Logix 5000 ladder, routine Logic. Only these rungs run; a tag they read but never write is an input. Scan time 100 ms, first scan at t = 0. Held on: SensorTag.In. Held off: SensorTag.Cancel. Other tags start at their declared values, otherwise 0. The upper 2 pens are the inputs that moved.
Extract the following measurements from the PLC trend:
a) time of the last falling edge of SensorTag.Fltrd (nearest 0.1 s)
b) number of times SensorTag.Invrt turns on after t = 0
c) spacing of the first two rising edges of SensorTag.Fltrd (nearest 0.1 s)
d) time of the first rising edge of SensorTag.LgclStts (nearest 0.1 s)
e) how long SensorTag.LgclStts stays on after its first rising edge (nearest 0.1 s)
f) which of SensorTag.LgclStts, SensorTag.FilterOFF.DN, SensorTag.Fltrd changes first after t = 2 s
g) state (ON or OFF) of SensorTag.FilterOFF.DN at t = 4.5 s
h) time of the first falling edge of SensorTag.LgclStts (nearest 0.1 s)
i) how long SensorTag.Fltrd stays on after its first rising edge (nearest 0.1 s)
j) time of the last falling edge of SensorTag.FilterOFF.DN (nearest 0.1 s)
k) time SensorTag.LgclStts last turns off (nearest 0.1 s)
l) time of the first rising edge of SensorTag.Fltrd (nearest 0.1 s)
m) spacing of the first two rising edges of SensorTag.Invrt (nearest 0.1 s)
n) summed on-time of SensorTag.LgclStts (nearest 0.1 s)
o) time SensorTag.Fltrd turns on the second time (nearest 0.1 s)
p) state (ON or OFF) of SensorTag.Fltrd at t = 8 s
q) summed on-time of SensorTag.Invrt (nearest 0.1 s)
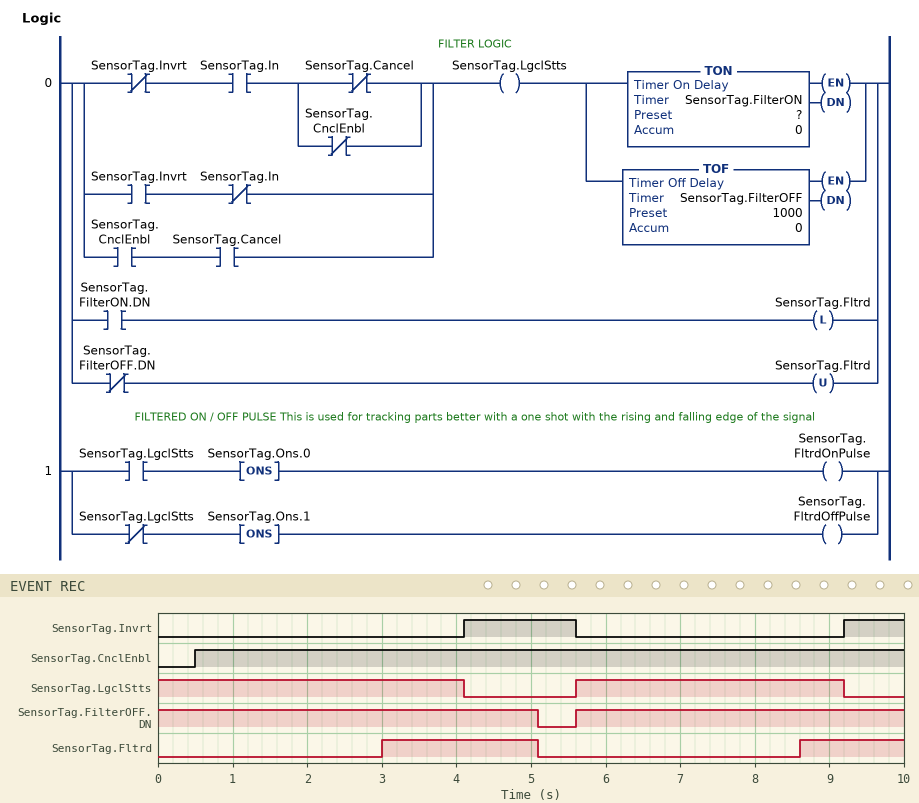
5.1 s
2
5.6 s
5.6 s
3.6 s
SensorTag.Fltrd
ON
4.1 s
2.1 s
5.1 s
9.2 s
3.0 s
5.1 s
7.7 s
8.6 s
OFF
2.3 s
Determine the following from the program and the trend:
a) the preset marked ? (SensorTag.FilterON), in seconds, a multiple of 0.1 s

3.0 s
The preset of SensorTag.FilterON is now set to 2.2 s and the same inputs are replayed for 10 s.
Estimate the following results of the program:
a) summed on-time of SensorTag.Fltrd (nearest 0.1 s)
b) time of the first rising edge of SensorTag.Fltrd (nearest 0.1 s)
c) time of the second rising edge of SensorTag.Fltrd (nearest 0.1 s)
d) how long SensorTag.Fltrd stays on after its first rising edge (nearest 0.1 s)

5.1 s
2.2 s
7.8 s
2.9 s
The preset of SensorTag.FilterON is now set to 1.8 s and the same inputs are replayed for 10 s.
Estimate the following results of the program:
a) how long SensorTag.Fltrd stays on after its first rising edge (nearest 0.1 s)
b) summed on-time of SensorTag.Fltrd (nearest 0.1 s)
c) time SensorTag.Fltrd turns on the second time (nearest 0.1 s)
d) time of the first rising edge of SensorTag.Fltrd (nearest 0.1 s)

3.3 s
5.9 s
7.4 s
1.8 s
